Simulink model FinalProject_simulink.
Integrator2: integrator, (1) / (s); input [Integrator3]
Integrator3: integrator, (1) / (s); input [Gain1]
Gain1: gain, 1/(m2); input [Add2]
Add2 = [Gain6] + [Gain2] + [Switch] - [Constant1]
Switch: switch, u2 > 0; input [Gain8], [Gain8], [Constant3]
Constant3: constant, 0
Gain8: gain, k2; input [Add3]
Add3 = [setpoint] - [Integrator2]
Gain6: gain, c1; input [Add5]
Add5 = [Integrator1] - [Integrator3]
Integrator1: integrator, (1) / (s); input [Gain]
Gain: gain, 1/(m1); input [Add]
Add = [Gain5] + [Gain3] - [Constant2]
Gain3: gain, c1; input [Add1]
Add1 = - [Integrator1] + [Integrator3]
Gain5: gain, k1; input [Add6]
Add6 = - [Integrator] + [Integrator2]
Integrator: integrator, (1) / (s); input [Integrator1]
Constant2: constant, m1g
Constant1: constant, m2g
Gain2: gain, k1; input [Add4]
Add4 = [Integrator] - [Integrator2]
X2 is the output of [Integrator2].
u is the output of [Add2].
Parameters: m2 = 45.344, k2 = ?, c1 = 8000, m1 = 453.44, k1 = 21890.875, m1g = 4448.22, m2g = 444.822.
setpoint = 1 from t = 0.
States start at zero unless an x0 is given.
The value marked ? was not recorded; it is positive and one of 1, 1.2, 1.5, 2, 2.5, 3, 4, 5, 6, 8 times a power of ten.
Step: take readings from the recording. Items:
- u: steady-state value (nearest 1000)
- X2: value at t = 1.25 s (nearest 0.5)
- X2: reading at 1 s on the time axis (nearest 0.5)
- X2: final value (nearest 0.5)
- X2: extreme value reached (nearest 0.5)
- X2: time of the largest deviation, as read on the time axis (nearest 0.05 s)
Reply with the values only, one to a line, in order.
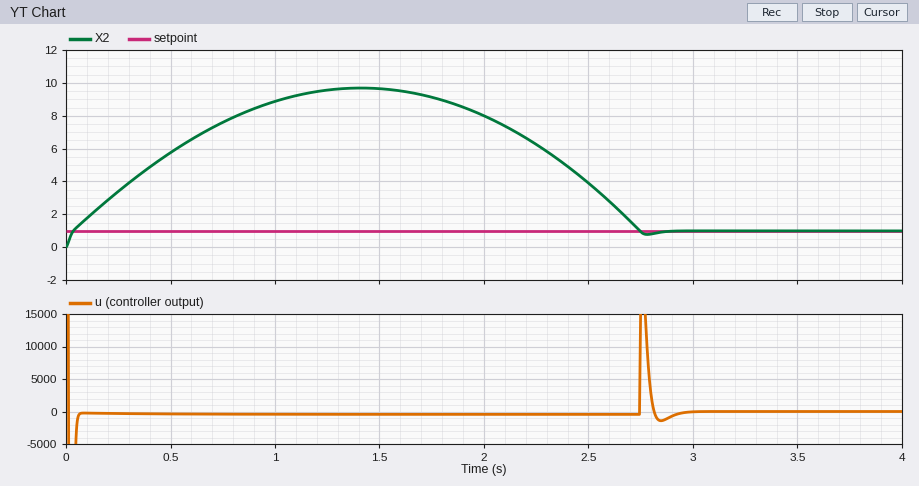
0
9.5
9.0
1.0
9.5
1.40 s
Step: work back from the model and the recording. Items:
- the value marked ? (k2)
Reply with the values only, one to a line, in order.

400000
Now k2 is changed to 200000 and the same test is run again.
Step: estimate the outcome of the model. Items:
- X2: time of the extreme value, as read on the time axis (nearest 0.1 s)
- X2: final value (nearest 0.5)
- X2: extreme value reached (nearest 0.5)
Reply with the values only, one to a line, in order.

1.2 s
1.0
6.5
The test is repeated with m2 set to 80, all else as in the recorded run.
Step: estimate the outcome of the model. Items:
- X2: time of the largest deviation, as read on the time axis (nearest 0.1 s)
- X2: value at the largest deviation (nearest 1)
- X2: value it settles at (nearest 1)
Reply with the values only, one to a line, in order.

1.6 s
12
1
